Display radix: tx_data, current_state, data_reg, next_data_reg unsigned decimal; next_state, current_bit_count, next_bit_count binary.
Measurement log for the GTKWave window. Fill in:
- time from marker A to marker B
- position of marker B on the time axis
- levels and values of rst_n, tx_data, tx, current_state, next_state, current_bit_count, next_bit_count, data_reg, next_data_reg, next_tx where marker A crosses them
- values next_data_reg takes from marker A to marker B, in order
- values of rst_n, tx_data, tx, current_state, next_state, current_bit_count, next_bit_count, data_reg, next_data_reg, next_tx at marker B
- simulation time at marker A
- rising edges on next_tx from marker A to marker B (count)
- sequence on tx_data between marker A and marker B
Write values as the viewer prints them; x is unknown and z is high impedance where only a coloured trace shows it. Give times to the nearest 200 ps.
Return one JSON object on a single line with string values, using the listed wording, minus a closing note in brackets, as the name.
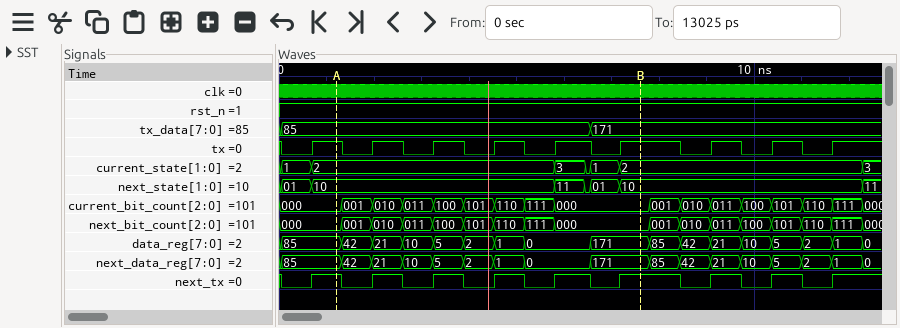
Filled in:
{"time from marker A to marker B": "6400 ps", "position of marker B on the time axis": "7600 ps", "levels and values of rst_n, tx_data, tx, current_state, next_state, current_bit_count, next_bit_count, data_reg, next_data_reg, next_tx where marker A crosses them": "rst_n=1, tx_data=85, tx=1, current_state=2, next_state=10, current_bit_count=000, next_bit_count=000, data_reg=85, next_data_reg=85, next_tx=1", "values next_data_reg takes from marker A to marker B, in order": "85, 42, 21, 10, 5, 2, 1, 0, 171", "values of rst_n, tx_data, tx, current_state, next_state, current_bit_count, next_bit_count, data_reg, next_data_reg, next_tx at marker B": "rst_n=1, tx_data=171, tx=1, current_state=2, next_state=10, current_bit_count=000, next_bit_count=000, data_reg=171, next_data_reg=171, next_tx=1", "simulation time at marker A": "1200 ps", "rising edges on next_tx from marker A to marker B": "5", "sequence on tx_data between marker A and marker B": "85, 171"}
